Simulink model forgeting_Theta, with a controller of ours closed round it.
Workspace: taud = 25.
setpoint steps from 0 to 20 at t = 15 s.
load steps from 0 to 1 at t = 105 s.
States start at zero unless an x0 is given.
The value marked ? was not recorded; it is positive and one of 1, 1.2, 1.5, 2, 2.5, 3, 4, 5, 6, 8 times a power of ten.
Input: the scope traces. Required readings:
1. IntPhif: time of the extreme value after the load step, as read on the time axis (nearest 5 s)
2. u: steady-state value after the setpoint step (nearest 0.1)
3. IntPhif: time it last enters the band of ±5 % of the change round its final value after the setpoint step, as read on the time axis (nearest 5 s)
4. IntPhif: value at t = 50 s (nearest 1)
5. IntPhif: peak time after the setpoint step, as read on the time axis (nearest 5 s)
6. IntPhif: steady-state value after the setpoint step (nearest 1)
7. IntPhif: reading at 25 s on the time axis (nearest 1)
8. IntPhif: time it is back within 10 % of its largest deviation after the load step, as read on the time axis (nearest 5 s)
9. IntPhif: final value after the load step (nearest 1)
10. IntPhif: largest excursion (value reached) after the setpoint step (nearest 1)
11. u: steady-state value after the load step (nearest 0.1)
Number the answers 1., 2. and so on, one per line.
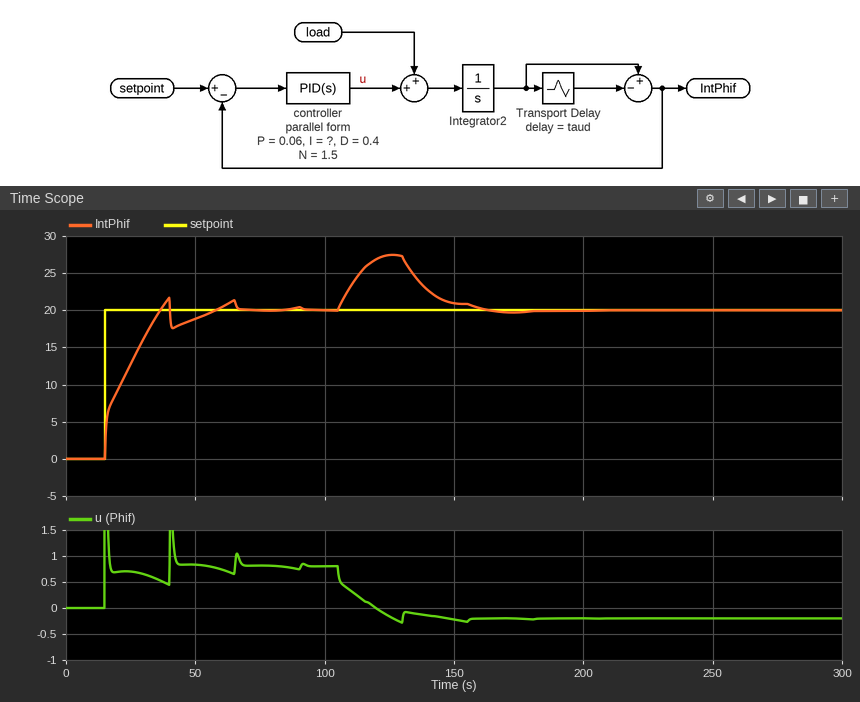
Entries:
1. 125 s
2. 0.8
3. 65 s
4. 19
5. 40 s
6. 20
7. 13
8. 155 s
9. 20
10. 22
11. -0.2
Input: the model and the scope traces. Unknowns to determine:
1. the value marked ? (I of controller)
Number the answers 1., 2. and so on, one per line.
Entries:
1. 0.005
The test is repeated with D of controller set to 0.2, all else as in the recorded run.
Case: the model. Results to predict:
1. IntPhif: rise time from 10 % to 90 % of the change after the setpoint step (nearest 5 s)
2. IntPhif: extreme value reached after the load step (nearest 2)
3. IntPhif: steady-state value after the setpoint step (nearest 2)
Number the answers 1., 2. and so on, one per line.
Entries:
1. 15 s
2. 28
3. 20
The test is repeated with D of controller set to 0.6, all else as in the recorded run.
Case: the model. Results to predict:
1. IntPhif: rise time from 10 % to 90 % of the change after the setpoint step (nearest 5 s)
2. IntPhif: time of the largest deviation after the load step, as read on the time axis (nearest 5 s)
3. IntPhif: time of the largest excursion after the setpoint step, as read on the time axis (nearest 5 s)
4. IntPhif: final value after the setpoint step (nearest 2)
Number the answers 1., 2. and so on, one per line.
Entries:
1. 20 s
2. 130 s
3. 65 s
4. 20
